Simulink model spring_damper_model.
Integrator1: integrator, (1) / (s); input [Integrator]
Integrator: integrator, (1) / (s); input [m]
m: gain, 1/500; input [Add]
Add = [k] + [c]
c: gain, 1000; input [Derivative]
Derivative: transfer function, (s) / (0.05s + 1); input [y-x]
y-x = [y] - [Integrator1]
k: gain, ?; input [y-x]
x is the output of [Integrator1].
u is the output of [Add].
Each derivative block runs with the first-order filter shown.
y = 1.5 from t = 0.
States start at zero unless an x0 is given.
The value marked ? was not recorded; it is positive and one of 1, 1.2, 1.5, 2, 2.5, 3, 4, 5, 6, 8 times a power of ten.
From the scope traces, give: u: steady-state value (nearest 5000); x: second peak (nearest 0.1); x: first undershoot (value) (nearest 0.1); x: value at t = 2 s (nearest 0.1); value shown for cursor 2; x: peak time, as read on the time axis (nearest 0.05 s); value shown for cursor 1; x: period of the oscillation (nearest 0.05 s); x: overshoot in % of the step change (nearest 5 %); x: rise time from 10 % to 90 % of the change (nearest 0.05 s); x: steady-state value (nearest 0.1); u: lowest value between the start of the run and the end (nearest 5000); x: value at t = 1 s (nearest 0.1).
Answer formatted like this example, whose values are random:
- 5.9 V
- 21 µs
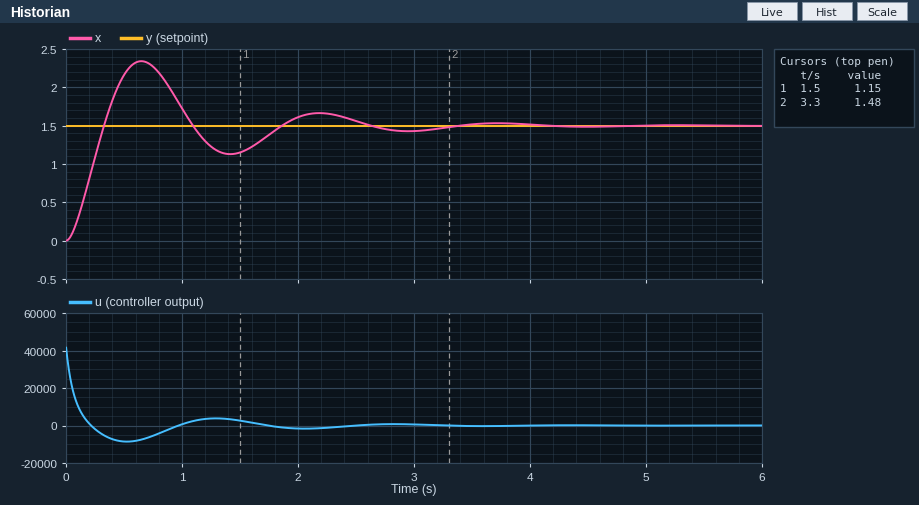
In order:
- 0
- 1.7
- 1.1
- 1.6
- 1.48
- 0.65 s
- 1.15
- 1.55 s
- 55 %
- 0.25 s
- 1.5
- -10000
- 1.7
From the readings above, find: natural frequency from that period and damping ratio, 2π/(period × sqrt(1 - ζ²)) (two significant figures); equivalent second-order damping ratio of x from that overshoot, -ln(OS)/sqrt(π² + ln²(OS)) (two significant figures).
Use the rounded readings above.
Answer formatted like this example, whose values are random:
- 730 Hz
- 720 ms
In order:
- 4.1 rad/s
- 0.19
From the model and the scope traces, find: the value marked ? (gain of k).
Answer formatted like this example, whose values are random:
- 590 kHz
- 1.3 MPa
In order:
- 8000
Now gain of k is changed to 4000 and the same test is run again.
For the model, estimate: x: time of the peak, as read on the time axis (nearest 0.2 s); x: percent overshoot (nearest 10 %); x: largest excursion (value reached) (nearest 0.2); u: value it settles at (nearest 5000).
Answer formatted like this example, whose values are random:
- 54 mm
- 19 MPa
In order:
- 0.8 s
- 40 %
- 2.2
- 0
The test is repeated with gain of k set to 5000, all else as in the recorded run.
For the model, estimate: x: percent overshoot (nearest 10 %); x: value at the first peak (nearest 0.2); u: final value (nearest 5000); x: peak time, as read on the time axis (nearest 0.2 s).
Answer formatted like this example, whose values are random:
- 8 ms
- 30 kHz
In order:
- 50 %
- 2.2
- 0
- 0.8 s
